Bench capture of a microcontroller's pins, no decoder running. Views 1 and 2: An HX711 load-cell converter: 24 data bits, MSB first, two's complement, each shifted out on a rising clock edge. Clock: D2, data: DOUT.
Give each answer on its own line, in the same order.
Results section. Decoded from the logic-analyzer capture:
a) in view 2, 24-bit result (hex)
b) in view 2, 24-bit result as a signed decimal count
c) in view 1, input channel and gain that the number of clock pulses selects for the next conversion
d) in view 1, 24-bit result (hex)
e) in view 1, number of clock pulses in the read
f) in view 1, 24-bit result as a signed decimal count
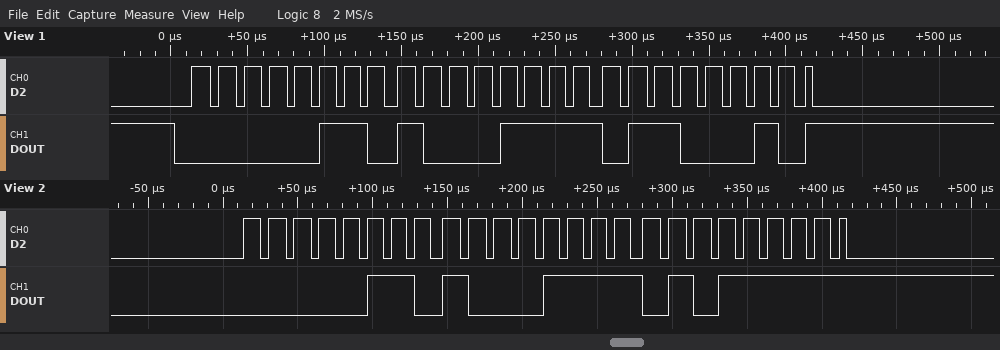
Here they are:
0x068F5F
429919
channel A, gain 128
0x068F62
25
429922
